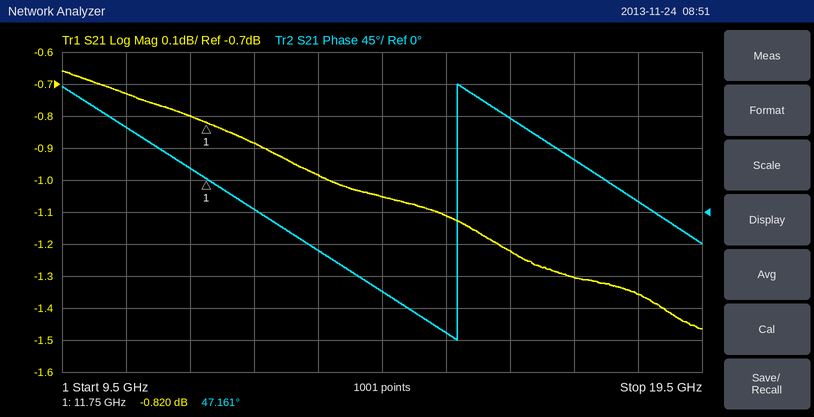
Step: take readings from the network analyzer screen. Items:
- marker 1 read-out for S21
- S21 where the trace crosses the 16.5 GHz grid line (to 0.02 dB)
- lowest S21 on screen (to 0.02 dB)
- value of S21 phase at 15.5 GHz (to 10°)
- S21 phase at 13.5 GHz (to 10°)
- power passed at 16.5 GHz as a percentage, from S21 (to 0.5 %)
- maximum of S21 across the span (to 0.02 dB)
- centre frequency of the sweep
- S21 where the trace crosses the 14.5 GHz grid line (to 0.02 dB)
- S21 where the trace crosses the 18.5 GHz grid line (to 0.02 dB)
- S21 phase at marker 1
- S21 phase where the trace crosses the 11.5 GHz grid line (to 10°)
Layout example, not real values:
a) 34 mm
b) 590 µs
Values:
a) -0.820 dB
b) -1.22 dB
c) -1.46 dB
d) -170°
e) -50°
f) 75.5 %
g) -0.66 dB
h) 14.5 GHz
i) -1.06 dB
j) -1.36 dB
k) 47.161°
l) 60°
